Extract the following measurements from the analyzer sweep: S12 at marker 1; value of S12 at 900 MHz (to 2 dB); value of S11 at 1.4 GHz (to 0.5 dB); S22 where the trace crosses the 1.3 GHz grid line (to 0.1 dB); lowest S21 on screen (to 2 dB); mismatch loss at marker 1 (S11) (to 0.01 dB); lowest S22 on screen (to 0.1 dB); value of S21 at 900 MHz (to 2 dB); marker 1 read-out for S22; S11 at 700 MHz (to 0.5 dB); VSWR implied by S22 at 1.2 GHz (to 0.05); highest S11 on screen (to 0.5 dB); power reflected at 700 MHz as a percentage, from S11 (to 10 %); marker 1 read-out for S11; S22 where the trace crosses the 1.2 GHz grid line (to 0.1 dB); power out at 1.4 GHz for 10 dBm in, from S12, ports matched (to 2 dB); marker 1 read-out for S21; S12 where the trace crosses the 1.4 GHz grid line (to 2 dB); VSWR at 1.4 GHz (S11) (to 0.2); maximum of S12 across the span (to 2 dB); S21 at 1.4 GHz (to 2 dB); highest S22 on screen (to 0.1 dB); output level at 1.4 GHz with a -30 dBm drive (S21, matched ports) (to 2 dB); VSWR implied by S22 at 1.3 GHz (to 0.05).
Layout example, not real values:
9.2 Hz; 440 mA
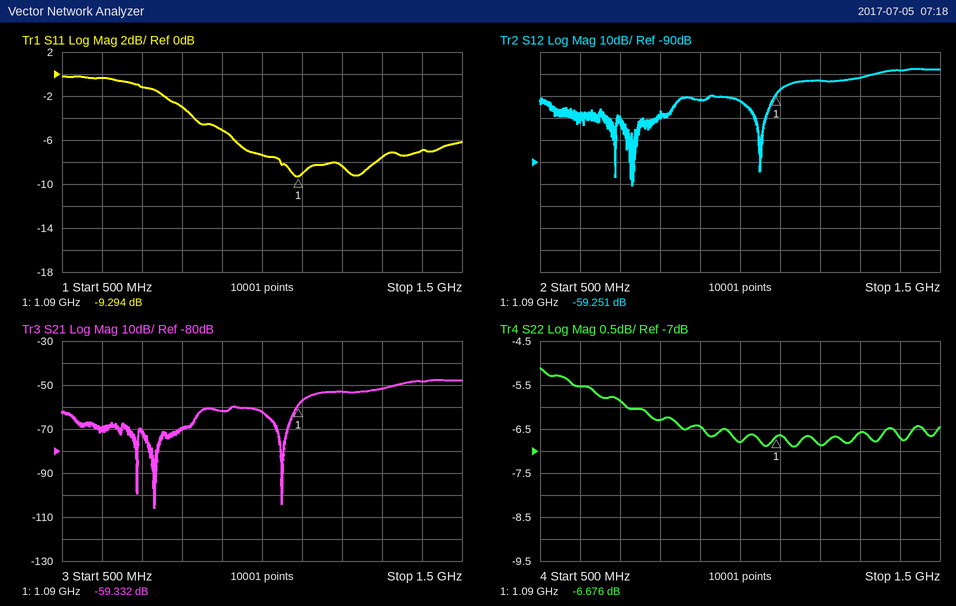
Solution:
-59.251 dB; -62 dB; -7.0 dB; -6.6 dB; -106 dB; 0.54 dB; -6.9 dB; -62 dB; -6.676 dB; -1.0 dB; 2.65; 0.0 dB; 80 %; -9.294 dB; -6.9 dB; -38 dBm; -59.332 dB; -48 dB; 2.6; -48 dB; -48 dB; -5.1 dB; -78 dBm; 2.75
